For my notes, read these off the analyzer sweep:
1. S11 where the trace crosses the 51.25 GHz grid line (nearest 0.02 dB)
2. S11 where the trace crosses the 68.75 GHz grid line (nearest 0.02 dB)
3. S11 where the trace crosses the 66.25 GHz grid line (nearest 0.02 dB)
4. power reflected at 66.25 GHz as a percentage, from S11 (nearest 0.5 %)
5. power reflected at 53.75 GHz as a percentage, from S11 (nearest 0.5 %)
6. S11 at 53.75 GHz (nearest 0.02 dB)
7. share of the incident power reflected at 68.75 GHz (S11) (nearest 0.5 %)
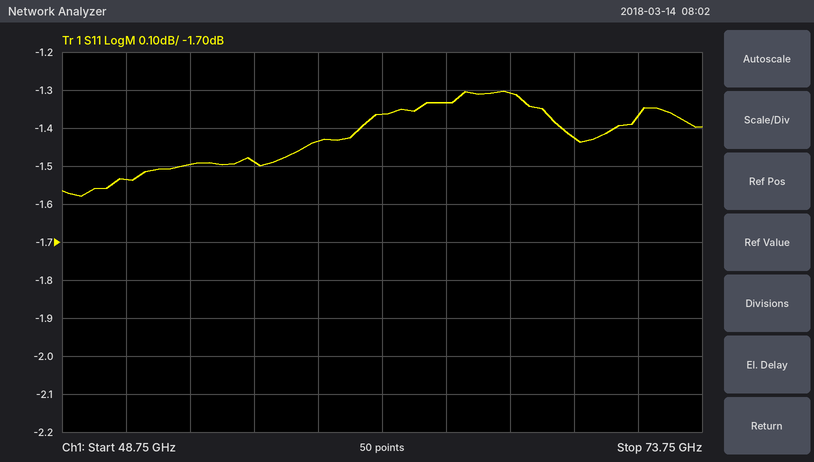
-1.54 dB
-1.42 dB
-1.30 dB
74.0 %
71.0 %
-1.50 dB
72.0 %
